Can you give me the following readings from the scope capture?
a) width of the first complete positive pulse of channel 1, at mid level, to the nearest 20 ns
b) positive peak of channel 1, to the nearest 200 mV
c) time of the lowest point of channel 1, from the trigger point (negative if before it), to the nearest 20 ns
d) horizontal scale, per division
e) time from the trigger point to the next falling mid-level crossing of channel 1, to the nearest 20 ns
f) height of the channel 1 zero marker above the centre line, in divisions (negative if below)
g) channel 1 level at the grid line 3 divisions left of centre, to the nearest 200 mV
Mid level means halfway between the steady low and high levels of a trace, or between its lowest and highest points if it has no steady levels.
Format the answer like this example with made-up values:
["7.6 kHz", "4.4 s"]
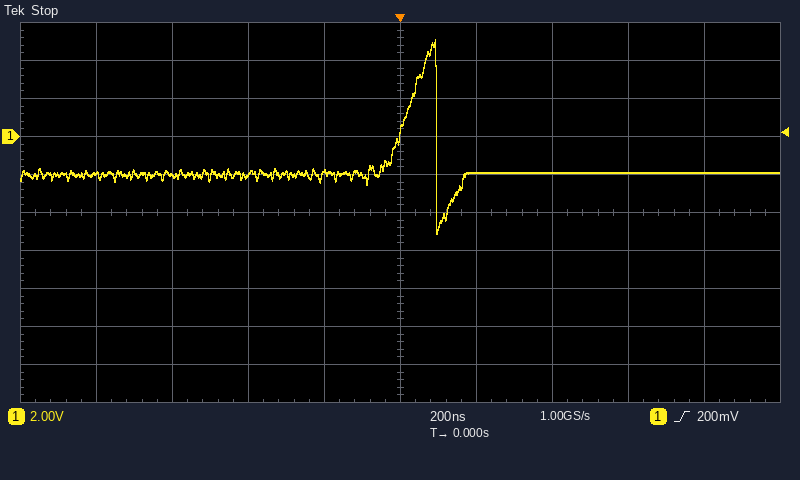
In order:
["100 ns", "5.2 V", "+100 ns", "200 ns", "100 ns", "+2.0 div", "-2.0 V"]
